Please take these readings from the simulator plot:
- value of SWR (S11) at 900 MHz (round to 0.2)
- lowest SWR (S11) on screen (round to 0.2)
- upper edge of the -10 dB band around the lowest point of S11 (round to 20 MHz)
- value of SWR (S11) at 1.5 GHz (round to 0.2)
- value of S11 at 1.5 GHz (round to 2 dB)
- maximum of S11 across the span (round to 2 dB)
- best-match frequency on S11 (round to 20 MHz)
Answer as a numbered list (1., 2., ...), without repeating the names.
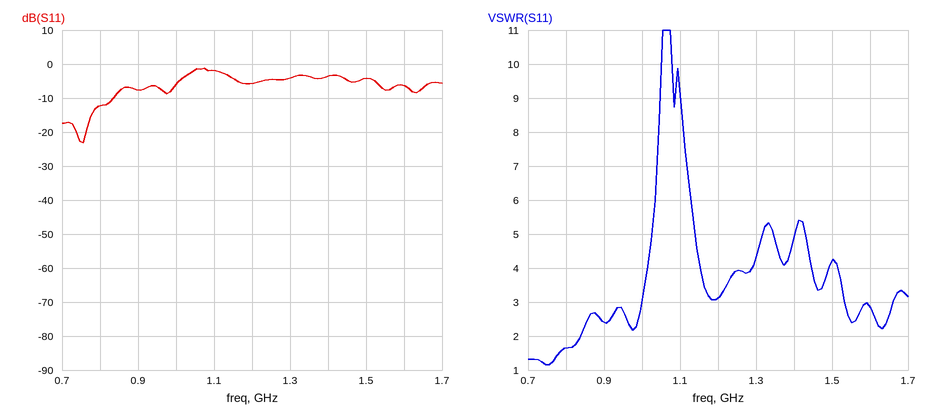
1. 2.4
2. 1.2
3. 840 MHz
4. 4.2
5. -4 dB
6. -2 dB
7. 760 MHz
